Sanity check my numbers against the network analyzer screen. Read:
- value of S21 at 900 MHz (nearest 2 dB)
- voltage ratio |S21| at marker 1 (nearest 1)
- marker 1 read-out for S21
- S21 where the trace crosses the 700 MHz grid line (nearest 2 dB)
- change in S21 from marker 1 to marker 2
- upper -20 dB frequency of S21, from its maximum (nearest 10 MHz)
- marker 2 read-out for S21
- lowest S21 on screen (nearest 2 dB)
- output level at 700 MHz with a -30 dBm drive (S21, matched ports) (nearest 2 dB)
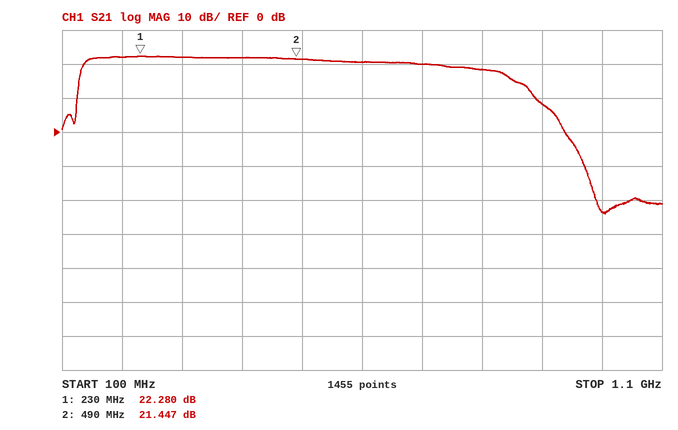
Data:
8 dB
13
22.280 dB
20 dB
-0.833 dB
930 MHz
21.447 dB
-24 dB
-10 dBm
